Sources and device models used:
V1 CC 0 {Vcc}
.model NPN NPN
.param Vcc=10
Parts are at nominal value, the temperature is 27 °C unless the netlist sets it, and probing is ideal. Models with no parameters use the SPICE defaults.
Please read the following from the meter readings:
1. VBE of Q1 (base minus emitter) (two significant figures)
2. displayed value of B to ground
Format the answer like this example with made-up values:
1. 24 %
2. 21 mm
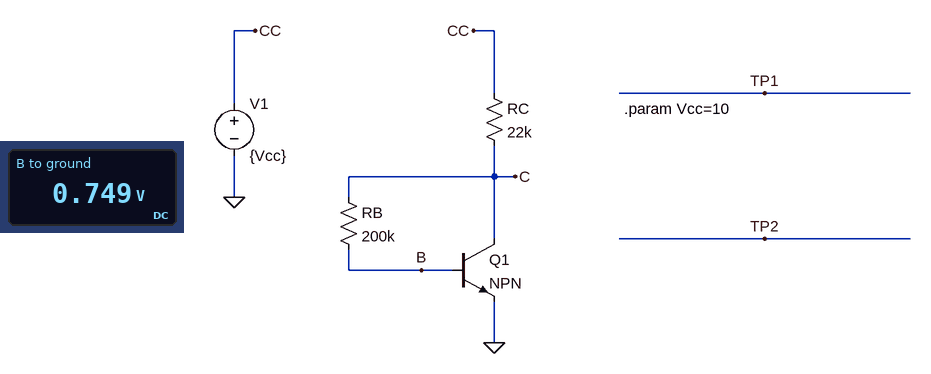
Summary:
1. 750 mV
2. 0.749 V
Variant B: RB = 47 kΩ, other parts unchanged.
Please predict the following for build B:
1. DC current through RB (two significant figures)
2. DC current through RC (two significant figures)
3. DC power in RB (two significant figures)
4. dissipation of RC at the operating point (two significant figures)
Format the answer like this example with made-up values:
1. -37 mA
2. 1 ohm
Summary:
1. 4.1 µA
2. 410 µA
3. 780 nW
4. 3.7 mW
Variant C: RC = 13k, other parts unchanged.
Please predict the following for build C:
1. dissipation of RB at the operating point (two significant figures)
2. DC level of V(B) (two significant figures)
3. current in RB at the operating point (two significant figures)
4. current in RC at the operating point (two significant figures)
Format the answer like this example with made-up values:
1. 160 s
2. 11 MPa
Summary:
1. 7.5 µW
2. 760 mV
3. 6.1 µA
4. 620 µA
